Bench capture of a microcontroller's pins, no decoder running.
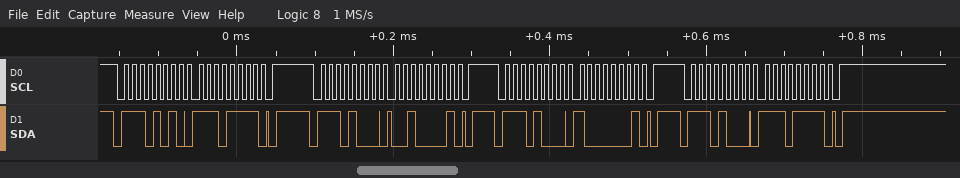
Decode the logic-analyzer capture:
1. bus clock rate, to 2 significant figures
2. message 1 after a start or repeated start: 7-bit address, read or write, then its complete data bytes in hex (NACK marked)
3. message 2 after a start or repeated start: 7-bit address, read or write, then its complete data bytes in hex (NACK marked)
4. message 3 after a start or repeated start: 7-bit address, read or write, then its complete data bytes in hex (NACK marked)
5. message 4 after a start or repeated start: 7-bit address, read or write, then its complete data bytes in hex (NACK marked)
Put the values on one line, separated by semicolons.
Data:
100 kHz; 0x75 write: EF; 0x74 write: 21; 0x74 write: 81; 0x74 write: EF
